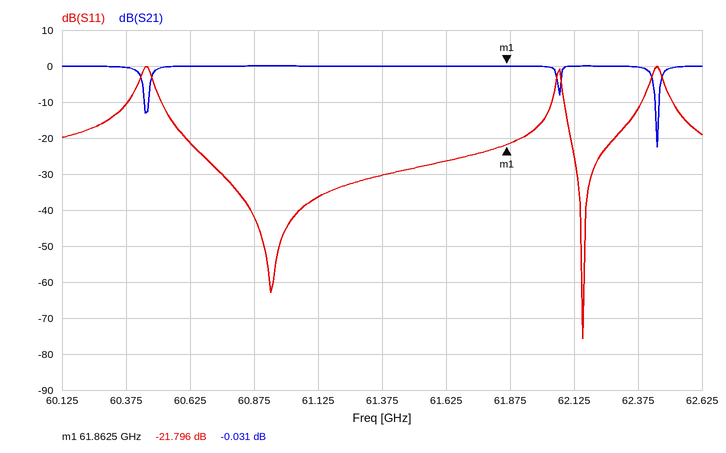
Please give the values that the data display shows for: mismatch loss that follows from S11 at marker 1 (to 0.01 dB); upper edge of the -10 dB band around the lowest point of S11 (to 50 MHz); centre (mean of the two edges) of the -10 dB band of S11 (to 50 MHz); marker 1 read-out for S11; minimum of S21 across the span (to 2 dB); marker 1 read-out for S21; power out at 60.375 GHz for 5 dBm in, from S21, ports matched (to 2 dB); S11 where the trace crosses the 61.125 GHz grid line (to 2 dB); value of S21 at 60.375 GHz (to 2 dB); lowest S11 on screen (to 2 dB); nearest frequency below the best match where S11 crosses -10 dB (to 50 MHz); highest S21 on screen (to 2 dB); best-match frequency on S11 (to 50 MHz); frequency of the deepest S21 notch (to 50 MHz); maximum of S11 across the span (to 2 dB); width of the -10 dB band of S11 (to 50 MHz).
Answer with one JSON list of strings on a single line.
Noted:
["0.03 dB", "62.40 GHz", "62.25 GHz", "-21.796 dB", "-22 dB", "-0.031 dB", "4 dBm", "-36 dB", "0 dB", "-76 dB", "62.10 GHz", "0 dB", "62.15 GHz", "62.45 GHz", "0 dB", "300 MHz"]
